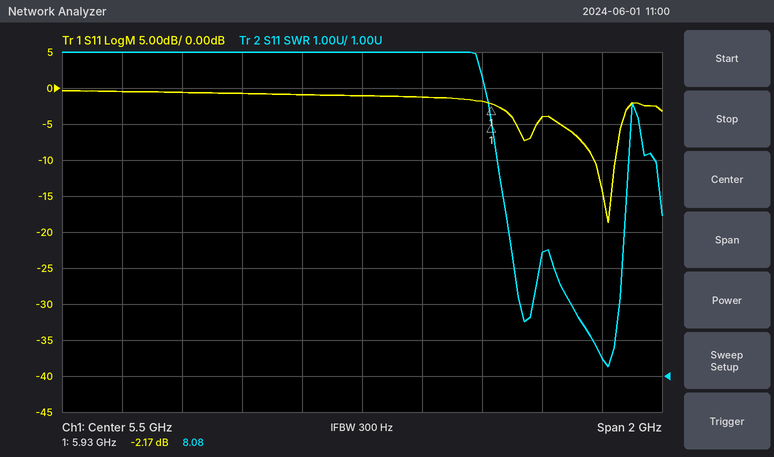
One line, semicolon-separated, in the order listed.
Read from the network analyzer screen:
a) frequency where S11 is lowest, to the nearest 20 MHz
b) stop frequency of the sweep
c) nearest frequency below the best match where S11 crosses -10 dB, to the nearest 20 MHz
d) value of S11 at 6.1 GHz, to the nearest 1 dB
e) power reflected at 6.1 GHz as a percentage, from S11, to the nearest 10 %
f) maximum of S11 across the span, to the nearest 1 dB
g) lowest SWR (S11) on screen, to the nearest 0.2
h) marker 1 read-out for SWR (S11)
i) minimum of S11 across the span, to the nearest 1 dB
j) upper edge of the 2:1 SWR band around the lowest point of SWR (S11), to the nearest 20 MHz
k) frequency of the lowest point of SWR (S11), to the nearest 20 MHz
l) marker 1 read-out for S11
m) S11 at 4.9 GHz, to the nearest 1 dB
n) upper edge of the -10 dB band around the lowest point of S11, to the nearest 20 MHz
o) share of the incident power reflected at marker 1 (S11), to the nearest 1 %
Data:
6.32 GHz; 6.5 GHz; 6.28 GHz; -4 dB; 40 %; 0 dB; 1.2; 8.08; -19 dB; 6.34 GHz; 6.32 GHz; -2.17 dB; -1 dB; 6.34 GHz; 61 %
